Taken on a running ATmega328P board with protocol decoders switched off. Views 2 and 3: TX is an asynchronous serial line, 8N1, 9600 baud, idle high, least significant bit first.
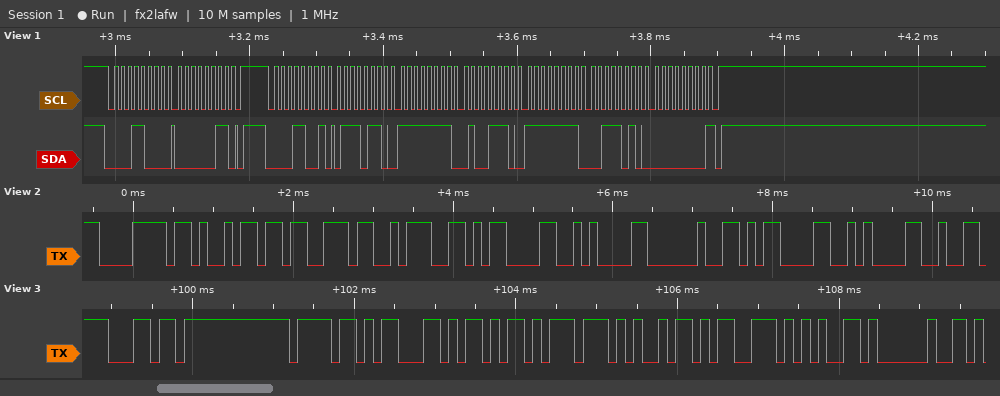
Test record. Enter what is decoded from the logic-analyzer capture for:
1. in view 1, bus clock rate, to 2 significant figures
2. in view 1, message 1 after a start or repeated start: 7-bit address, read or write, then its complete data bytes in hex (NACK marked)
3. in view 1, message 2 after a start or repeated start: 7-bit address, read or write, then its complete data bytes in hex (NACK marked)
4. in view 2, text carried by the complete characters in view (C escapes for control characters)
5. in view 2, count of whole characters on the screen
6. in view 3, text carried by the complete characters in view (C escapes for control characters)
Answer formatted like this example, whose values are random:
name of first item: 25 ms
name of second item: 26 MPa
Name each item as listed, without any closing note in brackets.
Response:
in view 1, bus clock rate, to 2 significant figures: 100 kHz
in view 1, message 1 after a start or repeated start: 7-bit address, read or write, then its complete data bytes in hex: 0x0C write: 03
in view 1, message 2 after a start or repeated start: 7-bit address, read or write, then its complete data bytes in hex: 0x0C read: 76 FF 4E FF 3A 00 NACK
in view 2, text carried by the complete characters in view: "xis:\r\n \r\n"
in view 2, count of whole characters on the screen: 9
in view 3, text carried by the complete characters in view: "lockwise "
